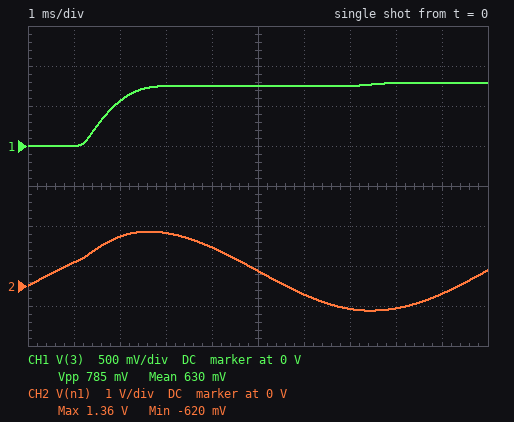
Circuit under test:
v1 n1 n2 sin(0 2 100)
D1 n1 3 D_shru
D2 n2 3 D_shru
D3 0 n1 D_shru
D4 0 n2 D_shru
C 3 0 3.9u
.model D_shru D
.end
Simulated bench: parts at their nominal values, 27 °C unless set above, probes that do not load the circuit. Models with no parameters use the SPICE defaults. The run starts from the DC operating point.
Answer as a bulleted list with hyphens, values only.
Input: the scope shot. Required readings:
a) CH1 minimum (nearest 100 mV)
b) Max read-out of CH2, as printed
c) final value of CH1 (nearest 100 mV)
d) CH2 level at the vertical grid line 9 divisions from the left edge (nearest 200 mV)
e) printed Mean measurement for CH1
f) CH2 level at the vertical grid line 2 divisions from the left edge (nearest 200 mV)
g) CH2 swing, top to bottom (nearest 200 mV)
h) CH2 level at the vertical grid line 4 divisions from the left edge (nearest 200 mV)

- 0 V
- 1.36 V
- 800 mV
- -200 mV
- 630 mV
- 1.2 V
- 2.0 V
- 1.0 V
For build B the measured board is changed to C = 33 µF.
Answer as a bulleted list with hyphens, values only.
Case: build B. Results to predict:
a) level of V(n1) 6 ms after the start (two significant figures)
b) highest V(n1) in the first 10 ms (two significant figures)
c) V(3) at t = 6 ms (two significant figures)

- -270 mV
- 1.3 V
- 640 mV
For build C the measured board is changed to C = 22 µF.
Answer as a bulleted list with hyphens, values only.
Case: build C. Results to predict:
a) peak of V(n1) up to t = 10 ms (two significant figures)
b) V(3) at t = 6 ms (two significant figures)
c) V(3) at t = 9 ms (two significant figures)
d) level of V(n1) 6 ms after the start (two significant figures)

- 1.3 V
- 660 mV
- 700 mV
- -260 mV
